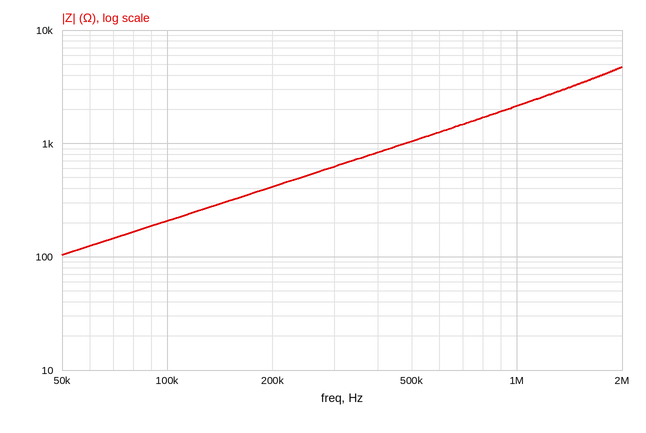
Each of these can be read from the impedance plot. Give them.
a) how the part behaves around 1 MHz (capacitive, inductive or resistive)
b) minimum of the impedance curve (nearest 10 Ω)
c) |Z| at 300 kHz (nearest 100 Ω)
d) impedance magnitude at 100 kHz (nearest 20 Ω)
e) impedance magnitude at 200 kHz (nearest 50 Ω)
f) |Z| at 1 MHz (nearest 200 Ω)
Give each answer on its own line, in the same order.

inductive
100 Ω
600 Ω
200 Ω
400 Ω
2.2 kΩ
